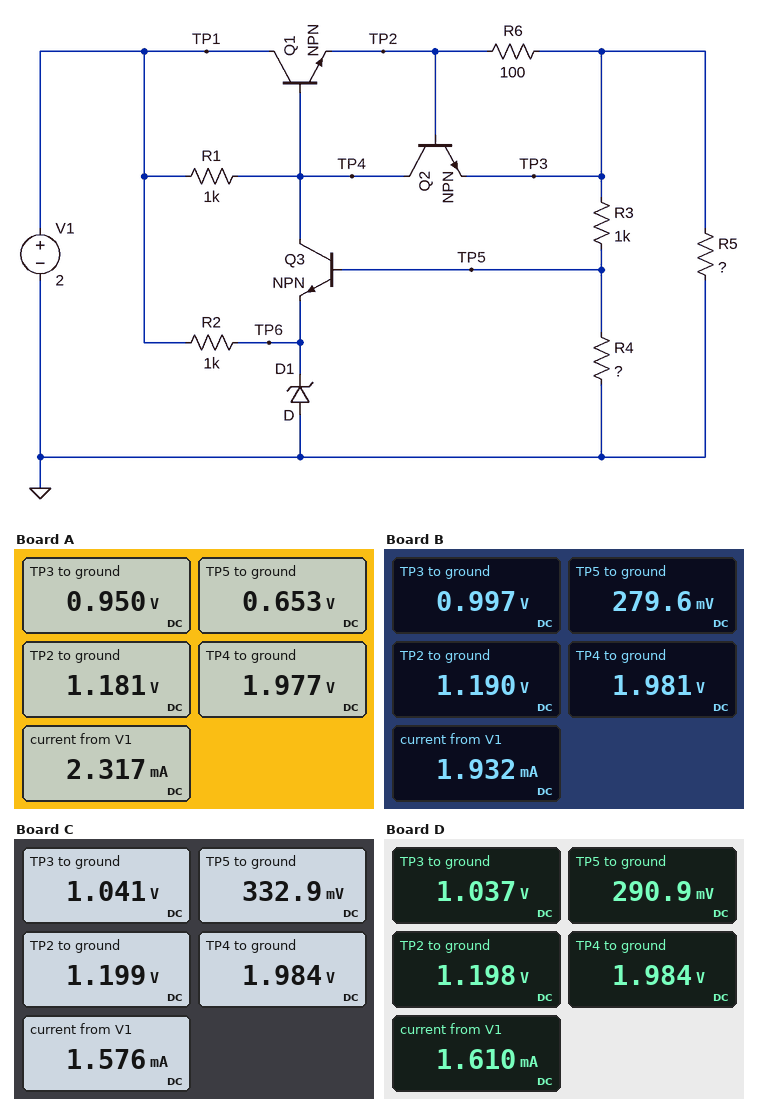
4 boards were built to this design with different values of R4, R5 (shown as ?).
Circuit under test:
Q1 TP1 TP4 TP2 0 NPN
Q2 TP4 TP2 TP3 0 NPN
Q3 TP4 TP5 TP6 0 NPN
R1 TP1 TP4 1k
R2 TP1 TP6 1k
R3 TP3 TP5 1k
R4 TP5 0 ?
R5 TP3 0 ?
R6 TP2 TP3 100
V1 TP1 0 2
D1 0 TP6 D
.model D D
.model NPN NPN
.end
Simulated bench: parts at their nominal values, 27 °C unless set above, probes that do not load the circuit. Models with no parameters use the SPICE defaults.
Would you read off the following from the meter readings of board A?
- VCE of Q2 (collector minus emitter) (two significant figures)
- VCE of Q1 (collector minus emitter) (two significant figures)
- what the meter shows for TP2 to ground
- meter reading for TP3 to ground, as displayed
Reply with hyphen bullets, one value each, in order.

- 1.0 V
- 820 mV
- 1.181 V
- 0.950 V
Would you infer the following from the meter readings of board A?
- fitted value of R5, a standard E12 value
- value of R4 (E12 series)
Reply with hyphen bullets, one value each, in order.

- 470 Ω
- 2.2 kΩ
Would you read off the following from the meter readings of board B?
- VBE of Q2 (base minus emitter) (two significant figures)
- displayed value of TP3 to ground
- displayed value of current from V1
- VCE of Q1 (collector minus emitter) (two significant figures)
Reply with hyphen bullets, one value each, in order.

- 190 mV
- 0.997 V
- 1.932 mA
- 810 mV
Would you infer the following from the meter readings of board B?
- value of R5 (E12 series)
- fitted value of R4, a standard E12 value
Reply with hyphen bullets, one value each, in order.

- 820 Ω
- 390 Ω
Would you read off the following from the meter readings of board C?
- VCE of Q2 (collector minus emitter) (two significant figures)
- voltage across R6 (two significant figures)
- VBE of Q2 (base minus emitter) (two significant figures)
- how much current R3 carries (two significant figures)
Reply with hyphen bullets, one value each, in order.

- 940 mV
- 160 mV
- 160 mV
- 710 µA
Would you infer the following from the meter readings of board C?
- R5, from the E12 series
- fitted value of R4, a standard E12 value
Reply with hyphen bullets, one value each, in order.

- 1.2 kΩ
- 470 Ω
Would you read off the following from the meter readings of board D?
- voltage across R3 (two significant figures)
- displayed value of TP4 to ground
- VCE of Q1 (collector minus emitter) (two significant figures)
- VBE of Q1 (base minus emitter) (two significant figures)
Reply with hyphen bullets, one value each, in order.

- 750 mV
- 1.984 V
- 800 mV
- 790 mV
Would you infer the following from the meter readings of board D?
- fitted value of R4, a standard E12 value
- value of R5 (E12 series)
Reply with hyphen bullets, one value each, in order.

- 390 Ω
- 1.2 kΩ
